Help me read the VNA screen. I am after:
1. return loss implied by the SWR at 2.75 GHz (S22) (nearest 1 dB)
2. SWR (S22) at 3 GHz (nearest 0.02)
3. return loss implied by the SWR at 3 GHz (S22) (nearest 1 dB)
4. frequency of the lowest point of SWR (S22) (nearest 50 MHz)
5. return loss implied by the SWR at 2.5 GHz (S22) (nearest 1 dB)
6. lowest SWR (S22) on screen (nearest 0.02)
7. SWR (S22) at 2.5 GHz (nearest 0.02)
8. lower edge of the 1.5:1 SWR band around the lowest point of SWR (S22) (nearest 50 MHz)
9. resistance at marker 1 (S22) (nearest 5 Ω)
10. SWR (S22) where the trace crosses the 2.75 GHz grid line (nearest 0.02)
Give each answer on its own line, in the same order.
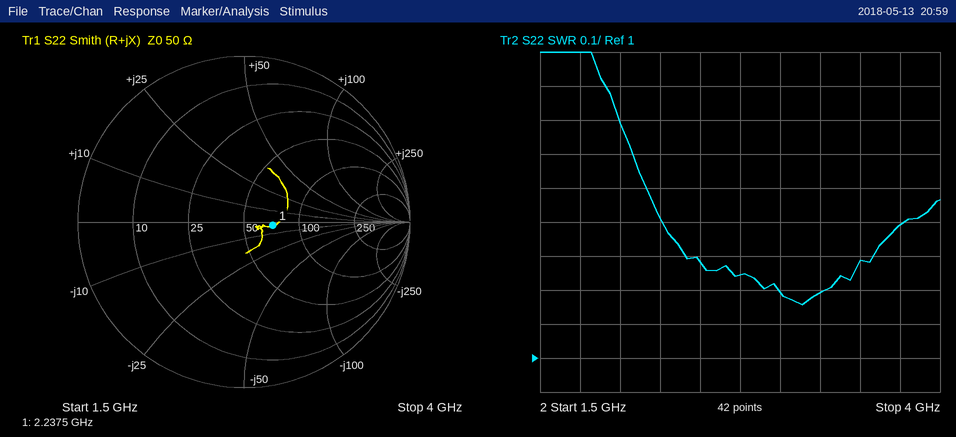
19 dB
1.20
21 dB
3.15 GHz
18 dB
1.16
1.28
2.15 GHz
70 Ω
1.24
